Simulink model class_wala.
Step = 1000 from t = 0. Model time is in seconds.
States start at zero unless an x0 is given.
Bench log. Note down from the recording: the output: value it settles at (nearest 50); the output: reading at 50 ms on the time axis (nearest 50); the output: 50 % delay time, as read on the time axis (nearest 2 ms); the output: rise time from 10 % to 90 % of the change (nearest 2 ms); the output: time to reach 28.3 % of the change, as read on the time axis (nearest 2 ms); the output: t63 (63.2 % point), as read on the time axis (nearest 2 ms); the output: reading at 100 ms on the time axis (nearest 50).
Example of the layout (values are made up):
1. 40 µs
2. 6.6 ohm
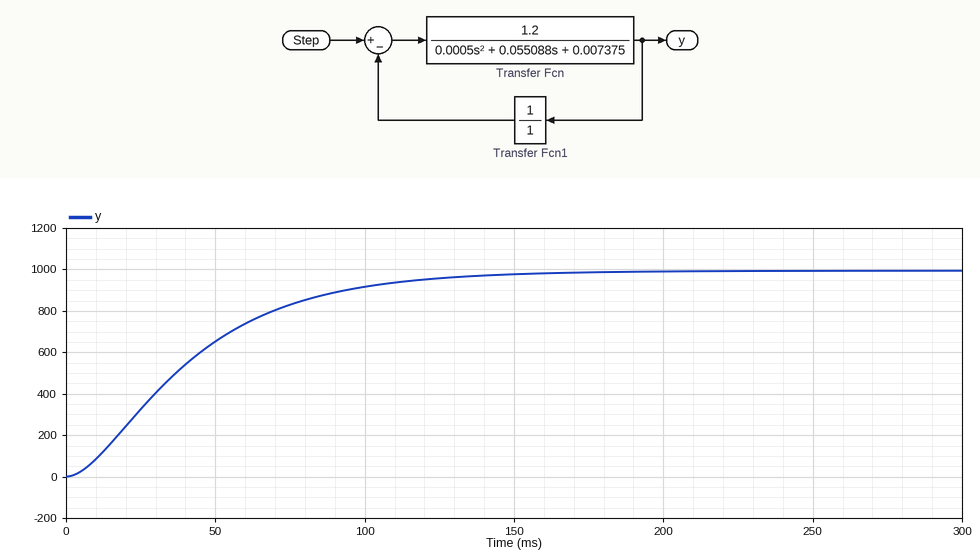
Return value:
1. 1000
2. 650
3. 36 ms
4. 80 ms
5. 22 ms
6. 48 ms
7. 900
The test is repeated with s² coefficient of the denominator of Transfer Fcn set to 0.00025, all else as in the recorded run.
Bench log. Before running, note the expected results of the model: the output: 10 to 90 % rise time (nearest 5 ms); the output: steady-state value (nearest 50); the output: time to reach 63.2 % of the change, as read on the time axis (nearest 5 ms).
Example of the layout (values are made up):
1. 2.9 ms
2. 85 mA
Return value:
1. 90 ms
2. 1000
3. 45 ms
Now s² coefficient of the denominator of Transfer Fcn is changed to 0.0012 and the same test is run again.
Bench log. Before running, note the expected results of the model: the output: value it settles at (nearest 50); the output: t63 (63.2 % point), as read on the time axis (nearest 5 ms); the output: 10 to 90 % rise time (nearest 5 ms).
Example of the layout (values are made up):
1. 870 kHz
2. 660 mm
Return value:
1. 1000
2. 55 ms
3. 70 ms
